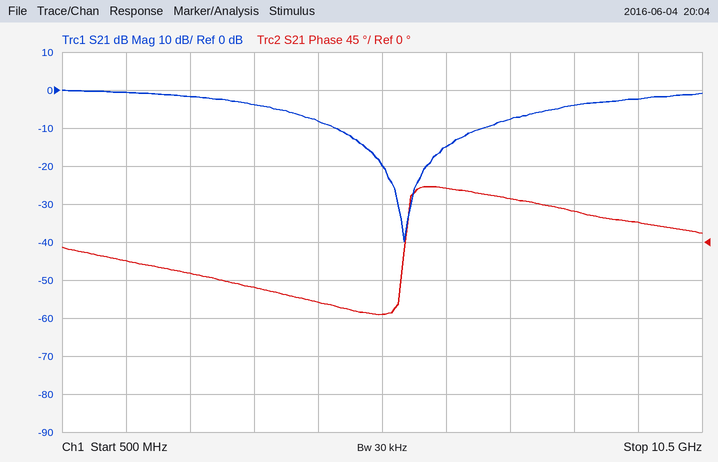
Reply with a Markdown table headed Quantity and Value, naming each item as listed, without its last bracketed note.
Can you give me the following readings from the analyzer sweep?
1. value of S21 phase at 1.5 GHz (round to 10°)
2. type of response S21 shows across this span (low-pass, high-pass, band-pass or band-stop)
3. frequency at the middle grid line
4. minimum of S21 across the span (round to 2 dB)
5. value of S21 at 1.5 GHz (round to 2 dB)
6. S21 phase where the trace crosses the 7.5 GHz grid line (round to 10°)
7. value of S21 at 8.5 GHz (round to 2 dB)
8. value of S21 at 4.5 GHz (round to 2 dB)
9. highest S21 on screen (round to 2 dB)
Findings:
| Quantity | Value |
|---|---|
| value of S21 phase at 1.5 GHz | -20° |
| type of response S21 shows across this span | band-stop |
| frequency at the middle grid line | 5.5 GHz |
| minimum of S21 across the span | -40 dB |
| value of S21 at 1.5 GHz | 0 dB |
| S21 phase where the trace crosses the 7.5 GHz grid line | 50° |
| value of S21 at 8.5 GHz | -4 dB |
| value of S21 at 4.5 GHz | -8 dB |
| highest S21 on screen | 0 dB |
